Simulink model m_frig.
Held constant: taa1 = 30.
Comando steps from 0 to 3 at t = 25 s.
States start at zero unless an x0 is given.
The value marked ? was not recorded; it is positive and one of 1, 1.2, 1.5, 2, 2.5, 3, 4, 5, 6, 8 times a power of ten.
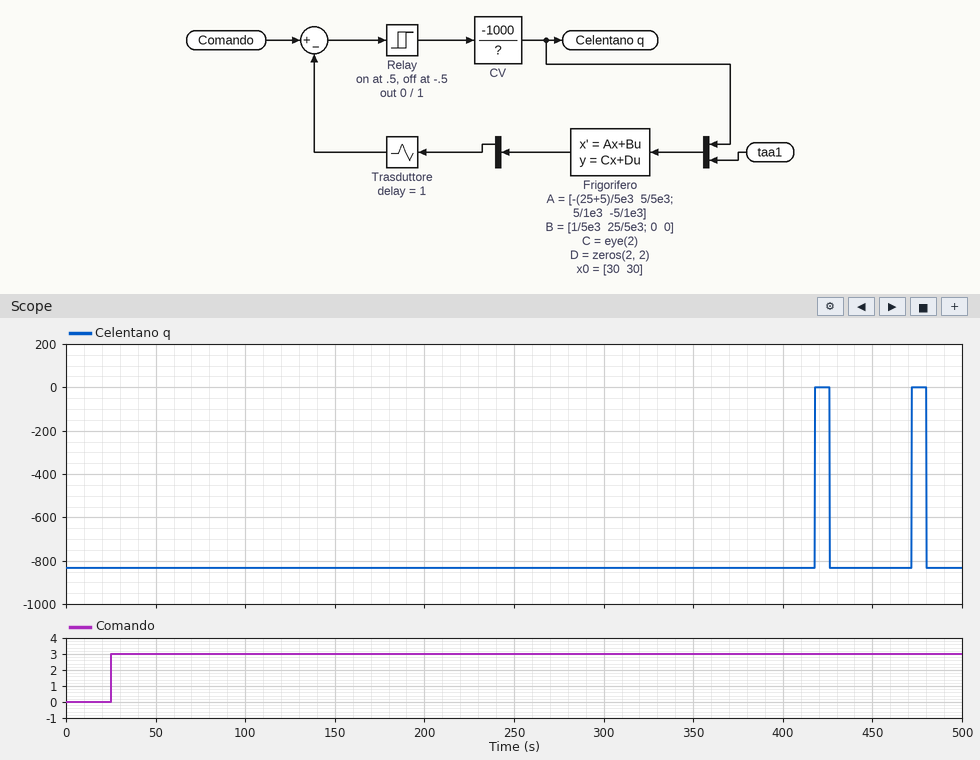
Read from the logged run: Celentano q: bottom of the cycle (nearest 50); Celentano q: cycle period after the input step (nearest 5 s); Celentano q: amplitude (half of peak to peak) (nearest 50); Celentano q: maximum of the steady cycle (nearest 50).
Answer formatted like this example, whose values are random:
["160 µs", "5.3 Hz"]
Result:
["-850", "55 s", "400", "0"]
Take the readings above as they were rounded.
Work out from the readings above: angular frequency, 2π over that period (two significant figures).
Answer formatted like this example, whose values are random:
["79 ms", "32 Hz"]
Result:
["0.11 rad/s"]
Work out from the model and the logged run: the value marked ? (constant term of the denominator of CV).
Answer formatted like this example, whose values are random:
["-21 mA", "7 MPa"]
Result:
["1.2"]
